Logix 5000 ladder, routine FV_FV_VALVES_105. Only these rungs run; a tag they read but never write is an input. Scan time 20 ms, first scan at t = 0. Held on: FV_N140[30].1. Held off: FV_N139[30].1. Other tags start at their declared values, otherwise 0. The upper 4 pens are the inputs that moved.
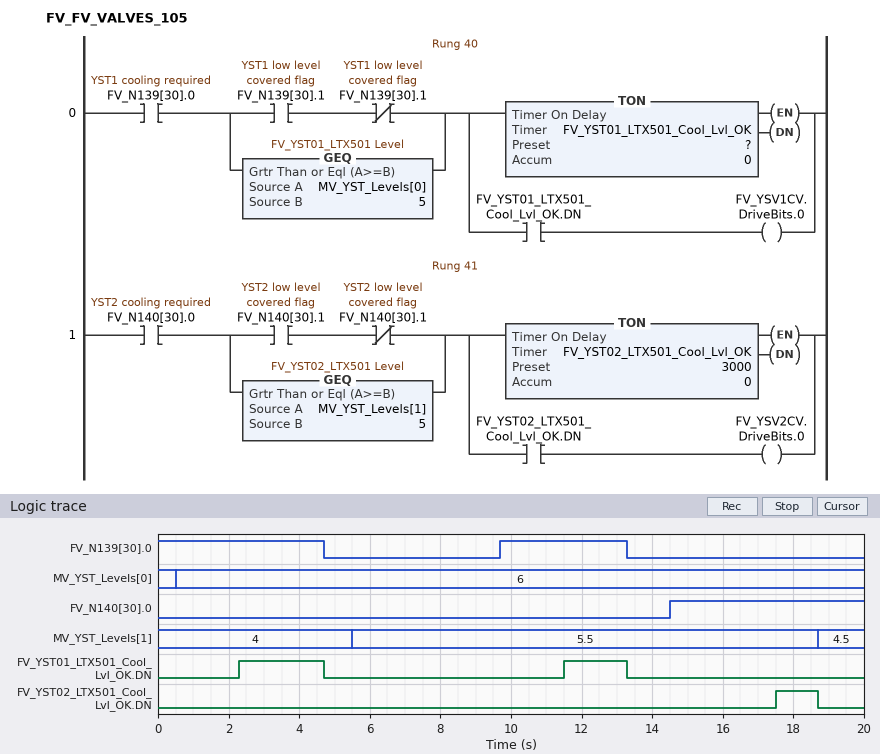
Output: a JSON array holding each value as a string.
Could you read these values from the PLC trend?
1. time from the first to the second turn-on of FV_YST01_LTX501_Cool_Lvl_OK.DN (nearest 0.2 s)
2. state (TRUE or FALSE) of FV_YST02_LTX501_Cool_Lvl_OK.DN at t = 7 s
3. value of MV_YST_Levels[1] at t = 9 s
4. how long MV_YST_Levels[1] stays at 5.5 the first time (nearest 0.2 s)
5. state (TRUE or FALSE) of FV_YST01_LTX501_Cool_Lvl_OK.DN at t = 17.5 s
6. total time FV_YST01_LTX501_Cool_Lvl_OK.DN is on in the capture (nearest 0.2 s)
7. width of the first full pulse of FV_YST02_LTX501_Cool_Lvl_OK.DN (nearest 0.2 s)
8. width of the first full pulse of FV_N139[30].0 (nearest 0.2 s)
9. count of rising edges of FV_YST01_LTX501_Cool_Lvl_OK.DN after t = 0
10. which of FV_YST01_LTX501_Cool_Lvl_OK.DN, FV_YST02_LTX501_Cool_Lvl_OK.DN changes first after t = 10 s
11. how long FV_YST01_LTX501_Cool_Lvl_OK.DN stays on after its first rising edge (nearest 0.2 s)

["9.2 s", "FALSE", "5.5", "13.2 s", "FALSE", "4.2 s", "1.2 s", "3.6 s", "2", "FV_YST01_LTX501_Cool_Lvl_OK.DN", "2.4 s"]
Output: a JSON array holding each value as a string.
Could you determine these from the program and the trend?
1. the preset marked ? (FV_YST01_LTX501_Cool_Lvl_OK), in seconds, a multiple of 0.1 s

["1.8 s"]
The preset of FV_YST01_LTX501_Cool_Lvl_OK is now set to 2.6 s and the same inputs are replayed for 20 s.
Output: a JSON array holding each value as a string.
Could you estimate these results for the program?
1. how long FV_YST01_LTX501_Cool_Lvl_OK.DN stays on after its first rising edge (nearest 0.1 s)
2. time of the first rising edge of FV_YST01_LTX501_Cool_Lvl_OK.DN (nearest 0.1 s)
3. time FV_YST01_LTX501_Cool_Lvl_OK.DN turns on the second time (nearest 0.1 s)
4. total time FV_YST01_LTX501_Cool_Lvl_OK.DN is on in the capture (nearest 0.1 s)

["1.6 s", "3.1 s", "12.3 s", "2.6 s"]
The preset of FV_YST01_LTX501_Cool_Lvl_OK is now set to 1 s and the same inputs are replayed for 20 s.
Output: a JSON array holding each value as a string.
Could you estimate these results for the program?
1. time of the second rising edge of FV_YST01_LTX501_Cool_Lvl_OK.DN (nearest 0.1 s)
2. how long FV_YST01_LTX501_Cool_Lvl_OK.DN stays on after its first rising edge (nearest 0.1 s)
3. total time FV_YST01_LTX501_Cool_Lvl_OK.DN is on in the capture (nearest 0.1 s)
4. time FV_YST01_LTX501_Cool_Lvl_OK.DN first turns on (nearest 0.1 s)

["10.7 s", "3.2 s", "5.8 s", "1.5 s"]
